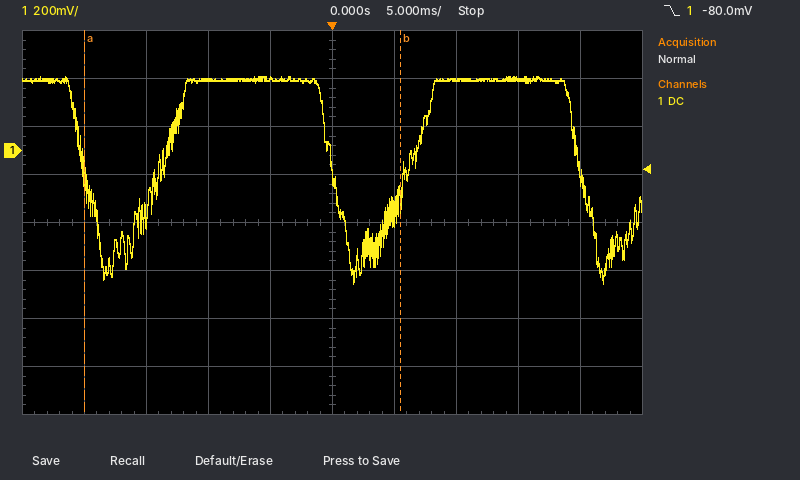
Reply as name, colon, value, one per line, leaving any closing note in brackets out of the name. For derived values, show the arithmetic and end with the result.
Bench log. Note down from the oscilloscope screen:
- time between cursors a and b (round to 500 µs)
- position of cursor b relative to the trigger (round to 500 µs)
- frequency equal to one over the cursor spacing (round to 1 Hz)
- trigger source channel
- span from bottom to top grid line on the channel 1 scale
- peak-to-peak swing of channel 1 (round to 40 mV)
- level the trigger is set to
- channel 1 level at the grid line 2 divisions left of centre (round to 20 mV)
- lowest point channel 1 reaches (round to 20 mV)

time between cursors a and b: 25.5 ms
position of cursor b relative to the trigger: +5.5 ms
frequency equal to one over the cursor spacing: 1 / 25.5 ms ≈ 39 Hz
trigger source channel: channel 1
span from bottom to top grid line on the channel 1 scale: 1.6 V
peak-to-peak swing of channel 1: 880 mV
level the trigger is set to: -80.0 mV
channel 1 level at the grid line 2 divisions left of centre: 300 mV
lowest point channel 1 reaches: -560 mV
